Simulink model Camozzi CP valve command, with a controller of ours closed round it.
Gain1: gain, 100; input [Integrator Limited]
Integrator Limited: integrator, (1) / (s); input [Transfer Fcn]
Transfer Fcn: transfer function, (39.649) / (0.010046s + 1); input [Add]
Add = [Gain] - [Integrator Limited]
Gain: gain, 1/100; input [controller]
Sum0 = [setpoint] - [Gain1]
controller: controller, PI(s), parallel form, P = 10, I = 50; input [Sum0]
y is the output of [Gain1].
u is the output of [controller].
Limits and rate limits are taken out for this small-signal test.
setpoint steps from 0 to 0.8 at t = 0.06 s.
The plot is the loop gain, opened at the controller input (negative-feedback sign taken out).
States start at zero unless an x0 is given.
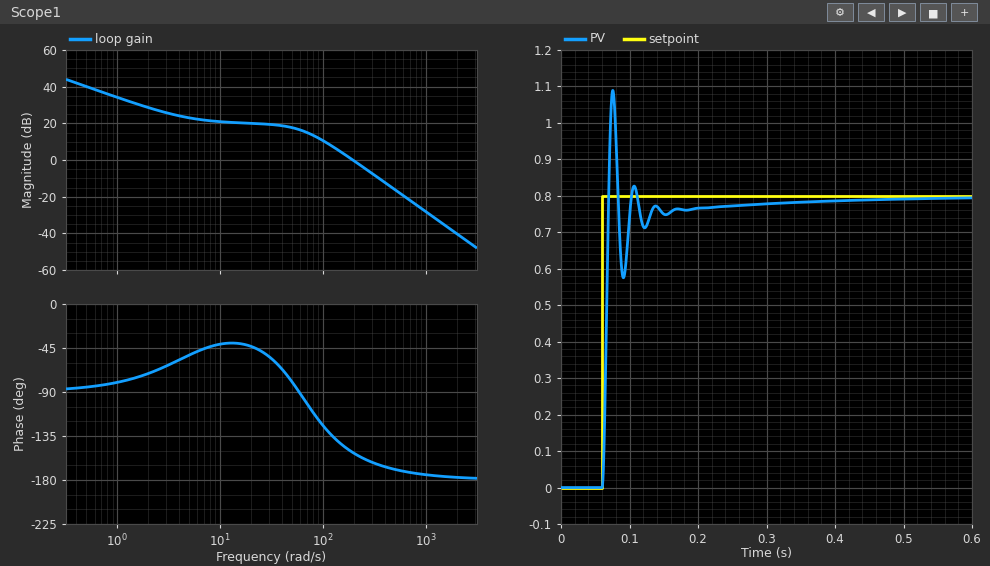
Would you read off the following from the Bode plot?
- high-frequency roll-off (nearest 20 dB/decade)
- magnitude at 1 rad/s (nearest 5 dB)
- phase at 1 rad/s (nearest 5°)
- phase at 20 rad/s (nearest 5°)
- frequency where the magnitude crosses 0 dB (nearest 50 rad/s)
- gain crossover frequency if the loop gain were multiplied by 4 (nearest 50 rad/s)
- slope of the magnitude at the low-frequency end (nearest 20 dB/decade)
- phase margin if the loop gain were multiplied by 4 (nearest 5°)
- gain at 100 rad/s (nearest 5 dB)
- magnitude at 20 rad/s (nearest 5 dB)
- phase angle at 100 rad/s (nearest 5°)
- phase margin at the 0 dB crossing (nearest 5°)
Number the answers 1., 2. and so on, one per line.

1. -40 dB/decade
2. 35 dB
3. -80°
4. -45°
5. 200 rad/s
6. 400 rad/s
7. -20 dB/decade
8. 15°
9. 10 dB
10. 20 dB
11. -125°
12. 30°
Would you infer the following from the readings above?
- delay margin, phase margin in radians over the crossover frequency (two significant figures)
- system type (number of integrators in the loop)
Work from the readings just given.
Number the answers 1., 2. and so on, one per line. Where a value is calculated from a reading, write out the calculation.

1. 30 × π / 180 / 200 = 0.0026 s
2. 1
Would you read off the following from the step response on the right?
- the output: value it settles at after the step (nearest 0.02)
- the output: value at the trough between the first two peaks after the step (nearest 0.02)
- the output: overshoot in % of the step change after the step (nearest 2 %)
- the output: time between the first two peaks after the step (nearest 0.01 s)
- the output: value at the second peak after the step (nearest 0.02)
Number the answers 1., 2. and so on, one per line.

1. 0.80
2. 0.58
3. 36 %
4. 0.03 s
5. 0.82
